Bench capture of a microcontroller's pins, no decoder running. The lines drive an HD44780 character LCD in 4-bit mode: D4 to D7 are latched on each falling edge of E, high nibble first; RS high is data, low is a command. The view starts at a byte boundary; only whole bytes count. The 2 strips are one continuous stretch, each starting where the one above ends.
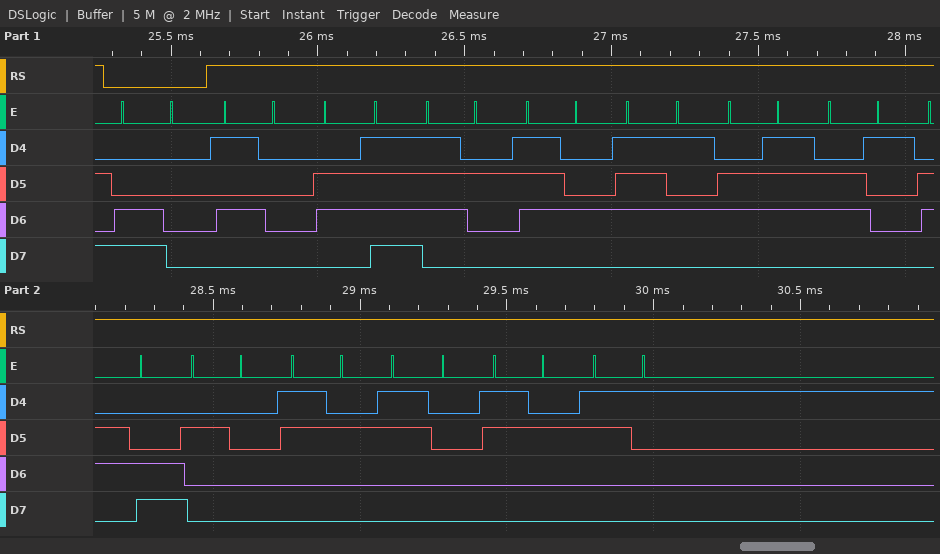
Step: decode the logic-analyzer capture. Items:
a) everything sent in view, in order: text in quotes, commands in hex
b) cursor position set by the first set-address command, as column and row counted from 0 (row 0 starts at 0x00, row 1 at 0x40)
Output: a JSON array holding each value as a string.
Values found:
["0xC0 \"Portugal 2021\"", "column 0, row 1"]
